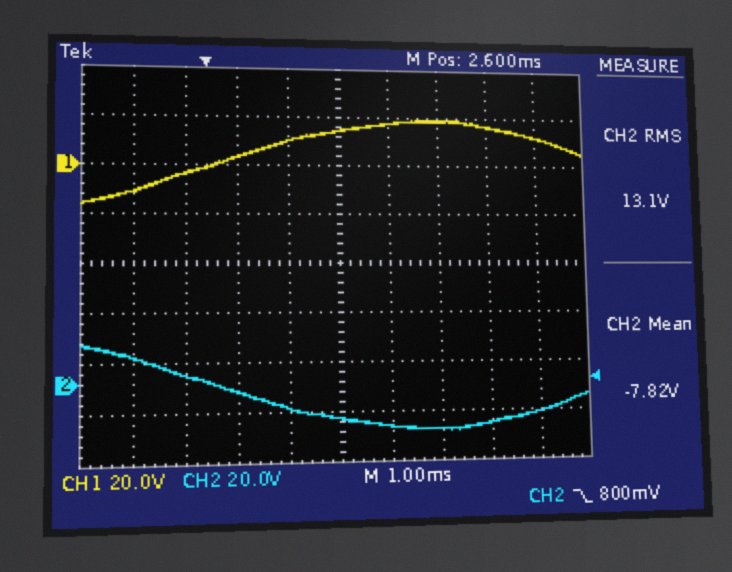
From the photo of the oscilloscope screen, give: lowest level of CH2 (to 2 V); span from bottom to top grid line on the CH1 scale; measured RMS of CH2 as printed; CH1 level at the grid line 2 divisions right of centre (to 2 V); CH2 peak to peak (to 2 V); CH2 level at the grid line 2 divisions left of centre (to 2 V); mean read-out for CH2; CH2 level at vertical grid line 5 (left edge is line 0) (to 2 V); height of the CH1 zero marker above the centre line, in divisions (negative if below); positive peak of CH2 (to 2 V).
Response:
-20 V
160 V
13.1 V
18 V
36 V
-4 V
-7.82 V
-14 V
+2.0 div
16 V
